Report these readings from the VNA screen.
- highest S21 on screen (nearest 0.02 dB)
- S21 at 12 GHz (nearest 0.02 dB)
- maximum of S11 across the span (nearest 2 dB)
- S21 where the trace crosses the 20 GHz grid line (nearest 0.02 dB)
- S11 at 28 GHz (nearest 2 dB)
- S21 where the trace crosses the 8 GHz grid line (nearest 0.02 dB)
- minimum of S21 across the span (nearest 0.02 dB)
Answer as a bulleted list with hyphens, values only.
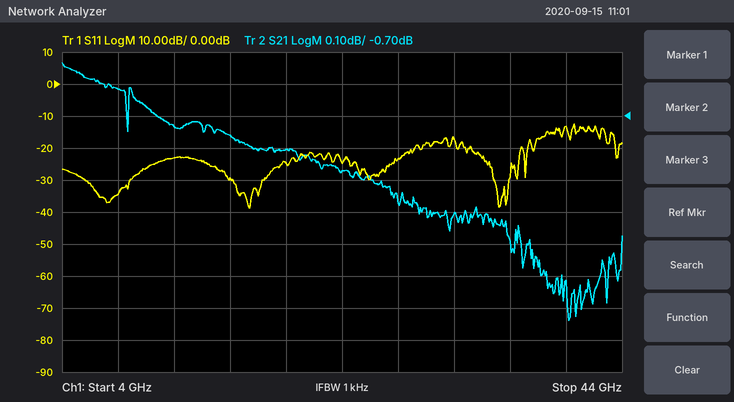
- -0.54 dB
- -0.74 dB
- -12 dB
- -0.80 dB
- -24 dB
- -0.62 dB
- -1.34 dB
